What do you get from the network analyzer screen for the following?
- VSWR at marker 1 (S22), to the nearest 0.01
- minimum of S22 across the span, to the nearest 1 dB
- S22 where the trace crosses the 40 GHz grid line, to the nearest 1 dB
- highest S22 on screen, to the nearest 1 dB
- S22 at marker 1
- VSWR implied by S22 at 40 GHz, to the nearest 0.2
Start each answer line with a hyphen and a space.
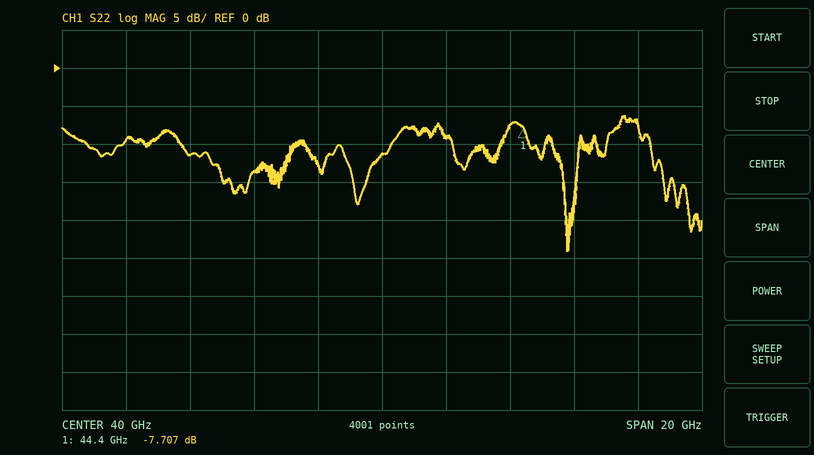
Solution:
- 2.40
- -24 dB
- -11 dB
- -6 dB
- -7.707 dB
- 1.8
